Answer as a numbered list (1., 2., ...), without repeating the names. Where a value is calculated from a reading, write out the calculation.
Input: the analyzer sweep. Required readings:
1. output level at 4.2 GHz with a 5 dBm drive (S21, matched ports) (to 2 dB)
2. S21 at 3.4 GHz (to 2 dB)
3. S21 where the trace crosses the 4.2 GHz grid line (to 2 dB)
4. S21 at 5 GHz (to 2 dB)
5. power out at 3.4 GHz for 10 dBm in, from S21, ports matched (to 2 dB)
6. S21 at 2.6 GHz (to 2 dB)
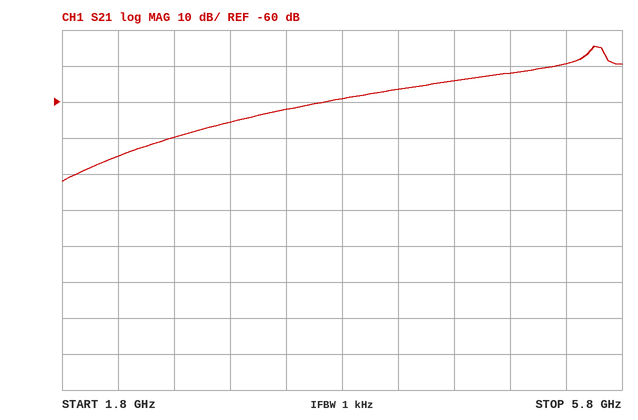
1. 5 dBm + (-56 dB) = -52 dBm
2. -62 dB
3. -56 dB
4. -52 dB
5. 10 dBm + (-62 dB) = -52 dBm
6. -70 dB
